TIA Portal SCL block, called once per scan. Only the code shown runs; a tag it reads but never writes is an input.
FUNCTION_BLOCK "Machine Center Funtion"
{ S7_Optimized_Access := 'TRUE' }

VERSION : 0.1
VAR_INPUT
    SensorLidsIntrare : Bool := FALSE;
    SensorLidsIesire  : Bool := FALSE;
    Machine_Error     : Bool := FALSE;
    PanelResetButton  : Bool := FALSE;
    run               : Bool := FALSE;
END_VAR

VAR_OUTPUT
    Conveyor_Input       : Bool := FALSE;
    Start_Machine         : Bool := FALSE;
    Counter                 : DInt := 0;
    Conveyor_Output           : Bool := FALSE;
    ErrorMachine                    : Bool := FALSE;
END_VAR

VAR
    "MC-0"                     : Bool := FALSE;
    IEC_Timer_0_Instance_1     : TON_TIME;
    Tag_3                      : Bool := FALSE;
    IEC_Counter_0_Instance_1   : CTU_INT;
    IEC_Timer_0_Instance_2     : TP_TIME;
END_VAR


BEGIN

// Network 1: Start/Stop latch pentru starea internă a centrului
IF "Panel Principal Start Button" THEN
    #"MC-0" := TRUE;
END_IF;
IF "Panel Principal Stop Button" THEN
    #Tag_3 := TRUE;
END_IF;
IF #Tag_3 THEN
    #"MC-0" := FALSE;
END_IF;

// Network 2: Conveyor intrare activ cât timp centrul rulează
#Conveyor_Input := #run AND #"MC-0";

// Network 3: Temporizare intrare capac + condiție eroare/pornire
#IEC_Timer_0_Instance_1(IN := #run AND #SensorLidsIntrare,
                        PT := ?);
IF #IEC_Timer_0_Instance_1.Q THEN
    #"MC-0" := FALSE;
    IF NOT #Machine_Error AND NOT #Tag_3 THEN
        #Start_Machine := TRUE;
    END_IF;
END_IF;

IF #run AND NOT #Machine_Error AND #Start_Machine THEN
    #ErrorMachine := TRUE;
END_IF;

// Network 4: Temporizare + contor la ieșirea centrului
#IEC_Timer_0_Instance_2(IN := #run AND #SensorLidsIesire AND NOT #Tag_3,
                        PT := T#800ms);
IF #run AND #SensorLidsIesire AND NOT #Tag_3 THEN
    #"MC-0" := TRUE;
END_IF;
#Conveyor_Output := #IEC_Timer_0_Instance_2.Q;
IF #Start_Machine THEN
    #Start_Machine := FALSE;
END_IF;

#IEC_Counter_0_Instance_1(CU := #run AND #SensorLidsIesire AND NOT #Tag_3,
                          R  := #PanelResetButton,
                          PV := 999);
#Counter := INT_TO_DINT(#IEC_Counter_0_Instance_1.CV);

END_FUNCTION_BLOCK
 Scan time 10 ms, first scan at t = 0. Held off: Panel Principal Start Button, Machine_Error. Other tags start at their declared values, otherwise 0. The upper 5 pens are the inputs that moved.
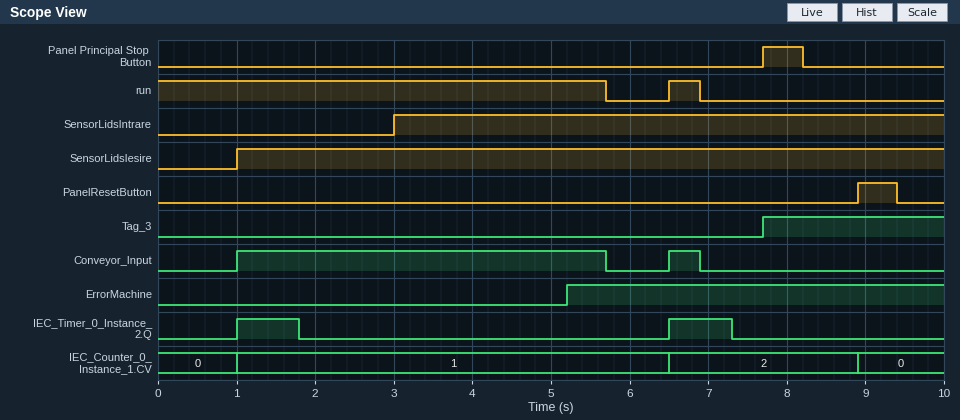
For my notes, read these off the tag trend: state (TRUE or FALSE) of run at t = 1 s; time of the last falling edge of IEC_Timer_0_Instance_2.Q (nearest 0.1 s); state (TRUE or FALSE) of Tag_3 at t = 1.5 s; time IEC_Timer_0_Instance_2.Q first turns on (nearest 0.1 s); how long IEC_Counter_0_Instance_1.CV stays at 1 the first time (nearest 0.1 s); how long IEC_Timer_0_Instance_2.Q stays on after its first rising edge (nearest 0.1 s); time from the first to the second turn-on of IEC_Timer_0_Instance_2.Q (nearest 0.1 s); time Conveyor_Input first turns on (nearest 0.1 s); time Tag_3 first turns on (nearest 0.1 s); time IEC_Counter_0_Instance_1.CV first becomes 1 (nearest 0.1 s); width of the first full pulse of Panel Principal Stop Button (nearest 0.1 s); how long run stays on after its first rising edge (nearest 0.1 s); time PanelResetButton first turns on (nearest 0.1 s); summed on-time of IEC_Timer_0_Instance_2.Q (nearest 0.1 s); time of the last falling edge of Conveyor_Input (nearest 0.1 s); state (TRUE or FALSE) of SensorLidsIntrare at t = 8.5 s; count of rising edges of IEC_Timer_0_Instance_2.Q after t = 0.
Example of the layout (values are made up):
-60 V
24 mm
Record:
TRUE
7.3 s
FALSE
1.0 s
5.5 s
0.8 s
5.5 s
1.0 s
7.7 s
1.0 s
0.5 s
0.4 s
8.9 s
1.6 s
6.9 s
TRUE
2
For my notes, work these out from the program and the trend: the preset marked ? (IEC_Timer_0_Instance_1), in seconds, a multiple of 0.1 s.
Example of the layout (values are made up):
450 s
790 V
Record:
2.2 s
